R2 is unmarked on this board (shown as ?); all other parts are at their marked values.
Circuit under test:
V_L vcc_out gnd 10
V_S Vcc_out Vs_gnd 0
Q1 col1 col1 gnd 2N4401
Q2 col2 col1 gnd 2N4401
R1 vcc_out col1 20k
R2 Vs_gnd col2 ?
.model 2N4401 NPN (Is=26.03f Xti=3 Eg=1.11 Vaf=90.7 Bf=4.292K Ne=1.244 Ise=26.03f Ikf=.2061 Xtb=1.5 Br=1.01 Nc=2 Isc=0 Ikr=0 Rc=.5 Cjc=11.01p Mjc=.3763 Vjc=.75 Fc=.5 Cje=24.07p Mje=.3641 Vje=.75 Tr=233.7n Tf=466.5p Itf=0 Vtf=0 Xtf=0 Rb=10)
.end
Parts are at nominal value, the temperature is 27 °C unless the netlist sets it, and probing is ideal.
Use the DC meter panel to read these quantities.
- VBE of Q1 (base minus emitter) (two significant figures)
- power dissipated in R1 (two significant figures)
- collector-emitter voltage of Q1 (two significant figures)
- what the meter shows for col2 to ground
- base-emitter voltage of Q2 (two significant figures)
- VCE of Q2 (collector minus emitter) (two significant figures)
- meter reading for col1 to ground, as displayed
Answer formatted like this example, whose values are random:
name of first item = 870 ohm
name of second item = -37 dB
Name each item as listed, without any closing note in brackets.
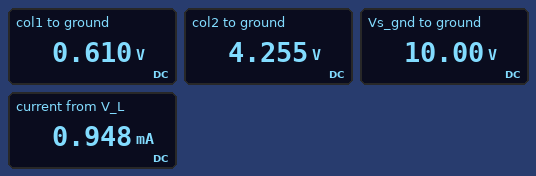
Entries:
VBE of Q1 (base minus emitter) = 610 mV
power dissipated in R1 = 4.4 mW
collector-emitter voltage of Q1 = 610 mV
what the meter shows for col2 to ground = 4.255 V
base-emitter voltage of Q2 = 610 mV
VCE of Q2 (collector minus emitter) = 4.3 V
meter reading for col1 to ground, as displayed = 0.610 V
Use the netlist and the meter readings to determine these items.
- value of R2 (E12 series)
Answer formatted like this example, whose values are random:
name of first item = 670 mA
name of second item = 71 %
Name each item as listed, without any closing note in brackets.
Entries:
value of R2 = 12 kΩ
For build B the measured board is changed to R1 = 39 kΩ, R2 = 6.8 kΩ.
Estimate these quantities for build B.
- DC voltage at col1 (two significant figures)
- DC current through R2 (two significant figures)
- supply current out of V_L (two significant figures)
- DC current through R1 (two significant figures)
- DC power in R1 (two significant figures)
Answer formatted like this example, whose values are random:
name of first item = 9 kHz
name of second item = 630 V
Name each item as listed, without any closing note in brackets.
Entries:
DC voltage at col1 = 590 mV
DC current through R2 = 260 µA
supply current out of V_L = 500 µA
DC current through R1 = 240 µA
DC power in R1 = 2.3 mW
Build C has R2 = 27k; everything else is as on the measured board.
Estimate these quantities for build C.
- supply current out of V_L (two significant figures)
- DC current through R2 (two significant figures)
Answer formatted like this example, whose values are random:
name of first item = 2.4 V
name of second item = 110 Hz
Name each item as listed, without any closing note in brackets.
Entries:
supply current out of V_L = 840 µA
DC current through R2 = 370 µA
